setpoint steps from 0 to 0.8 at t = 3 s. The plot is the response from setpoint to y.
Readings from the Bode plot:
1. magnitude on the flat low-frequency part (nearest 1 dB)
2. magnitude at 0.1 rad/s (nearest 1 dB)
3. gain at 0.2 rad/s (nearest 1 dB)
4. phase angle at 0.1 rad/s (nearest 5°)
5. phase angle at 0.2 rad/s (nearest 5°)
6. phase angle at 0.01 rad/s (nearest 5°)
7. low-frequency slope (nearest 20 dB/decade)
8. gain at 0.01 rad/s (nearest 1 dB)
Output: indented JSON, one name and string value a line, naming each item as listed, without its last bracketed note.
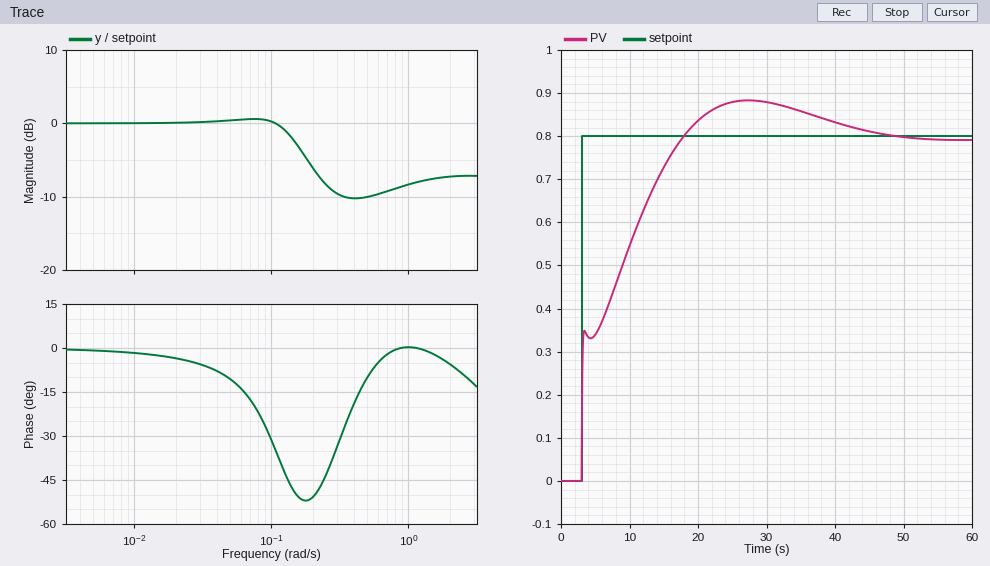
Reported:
{
  "magnitude on the flat low-frequency part": "0 dB",
  "magnitude at 0.1 rad/s": "0 dB",
  "gain at 0.2 rad/s": "-6 dB",
  "phase angle at 0.1 rad/s": "-30°",
  "phase angle at 0.2 rad/s": "-50°",
  "phase angle at 0.01 rad/s": "0°",
  "low-frequency slope": "0 dB/decade",
  "gain at 0.01 rad/s": "0 dB"
}
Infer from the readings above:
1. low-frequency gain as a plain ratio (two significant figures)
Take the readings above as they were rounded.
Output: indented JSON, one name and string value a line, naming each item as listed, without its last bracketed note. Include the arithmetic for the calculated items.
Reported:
{
  "low-frequency gain as a plain ratio": "10^(0 / 20) = 1.0"
}
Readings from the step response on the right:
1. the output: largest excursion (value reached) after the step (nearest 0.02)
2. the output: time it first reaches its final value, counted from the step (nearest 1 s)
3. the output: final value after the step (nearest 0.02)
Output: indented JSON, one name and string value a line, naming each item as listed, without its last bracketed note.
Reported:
{
  "the output: largest excursion (value reached) after the step": "0.88",
  "the output: time it first reaches its final value, counted from the step": "15 s",
  "the output: final value after the step": "0.80"
}
